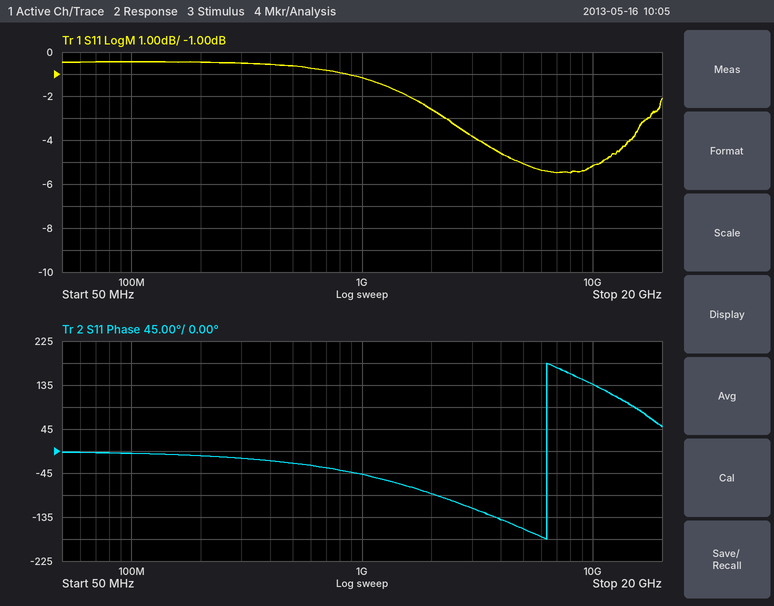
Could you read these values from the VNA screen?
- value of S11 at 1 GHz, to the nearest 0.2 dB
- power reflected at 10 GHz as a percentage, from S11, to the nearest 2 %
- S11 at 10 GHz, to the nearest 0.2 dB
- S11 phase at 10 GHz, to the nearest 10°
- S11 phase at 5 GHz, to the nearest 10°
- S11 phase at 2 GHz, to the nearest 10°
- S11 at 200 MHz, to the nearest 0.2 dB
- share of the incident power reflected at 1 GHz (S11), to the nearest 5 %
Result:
-1.2 dB
30 %
-5.2 dB
140°
-160°
-90°
-0.4 dB
75 %
